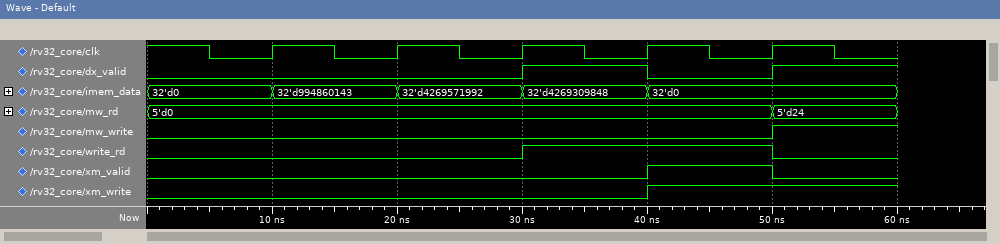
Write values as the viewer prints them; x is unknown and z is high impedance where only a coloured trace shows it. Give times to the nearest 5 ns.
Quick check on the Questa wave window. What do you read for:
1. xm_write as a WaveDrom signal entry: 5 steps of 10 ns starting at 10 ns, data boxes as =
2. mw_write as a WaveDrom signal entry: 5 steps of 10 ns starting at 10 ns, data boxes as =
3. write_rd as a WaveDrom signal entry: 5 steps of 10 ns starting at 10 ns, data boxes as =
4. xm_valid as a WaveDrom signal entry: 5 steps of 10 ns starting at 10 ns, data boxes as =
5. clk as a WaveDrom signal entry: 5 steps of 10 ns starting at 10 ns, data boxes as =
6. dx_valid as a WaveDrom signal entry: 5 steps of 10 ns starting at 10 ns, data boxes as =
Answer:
{name: 'xm_write', wave: '0..1.'}
{name: 'mw_write', wave: '0...1'}
{name: 'write_rd', wave: '0.1.0'}
{name: 'xm_valid', wave: '0..10'}
{name: 'clk', wave: 'p....'}
{name: 'dx_valid', wave: '0.101'}
